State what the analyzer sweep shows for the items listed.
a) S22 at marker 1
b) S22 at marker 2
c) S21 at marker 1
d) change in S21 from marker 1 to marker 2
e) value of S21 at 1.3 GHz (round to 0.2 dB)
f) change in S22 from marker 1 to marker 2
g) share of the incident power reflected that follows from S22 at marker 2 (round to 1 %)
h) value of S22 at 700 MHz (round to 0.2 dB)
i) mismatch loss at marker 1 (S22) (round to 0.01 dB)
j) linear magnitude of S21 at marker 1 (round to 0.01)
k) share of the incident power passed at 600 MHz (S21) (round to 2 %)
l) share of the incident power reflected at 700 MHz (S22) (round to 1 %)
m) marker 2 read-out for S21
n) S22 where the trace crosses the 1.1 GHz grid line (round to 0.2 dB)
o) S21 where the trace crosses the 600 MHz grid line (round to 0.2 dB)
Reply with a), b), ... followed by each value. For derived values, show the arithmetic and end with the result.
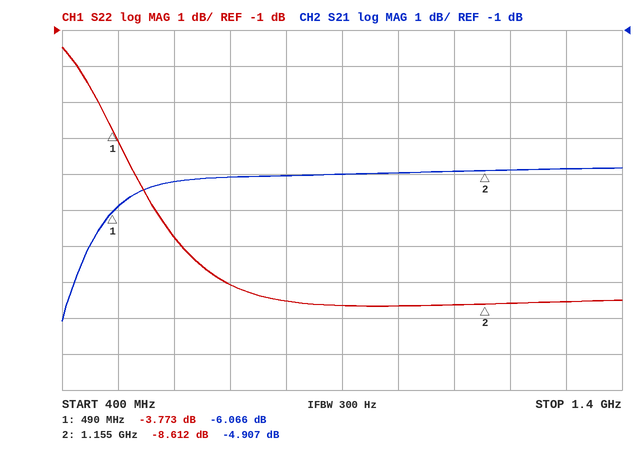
a) -3.773 dB
b) -8.612 dB
c) -6.066 dB
d) -4.907 − (-6.066) = 1.159 dB
e) -4.8 dB
f) -8.612 − (-3.773) = -4.839 dB
g) 10^(-8.612/10) ≈ 14 %
h) -8.0 dB
i) −10 log10(1 − 10^(-3.773/10)) ≈ 2.36 dB
j) 10^(-6.066/20) ≈ 0.50
k) 10^(-5.2/10) ≈ 30 %
l) 10^(-8/10) ≈ 16 %
m) -4.907 dB
n) -8.6 dB
o) -5.2 dB
